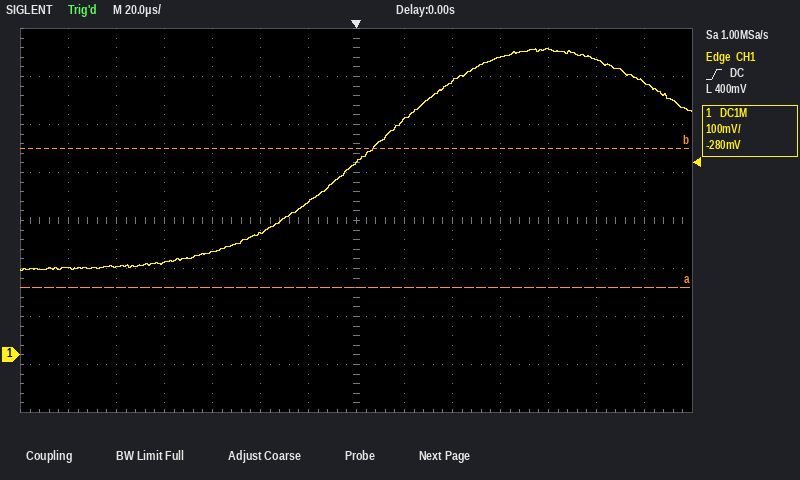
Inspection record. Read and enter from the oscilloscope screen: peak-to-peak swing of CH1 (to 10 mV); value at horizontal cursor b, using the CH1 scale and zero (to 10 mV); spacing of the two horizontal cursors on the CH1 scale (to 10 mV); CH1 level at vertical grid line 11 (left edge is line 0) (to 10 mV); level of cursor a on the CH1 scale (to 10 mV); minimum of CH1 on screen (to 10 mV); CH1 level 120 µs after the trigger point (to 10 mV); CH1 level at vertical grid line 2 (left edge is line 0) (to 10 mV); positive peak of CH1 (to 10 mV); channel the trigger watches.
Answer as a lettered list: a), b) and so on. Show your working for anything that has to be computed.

a) 640 mV − (180 mV) = 460 mV
b) 430 mV
c) 290 mV
d) 640 mV
e) 140 mV
f) 180 mV
g) 570 mV
h) 180 mV
i) 640 mV
j) CH1
